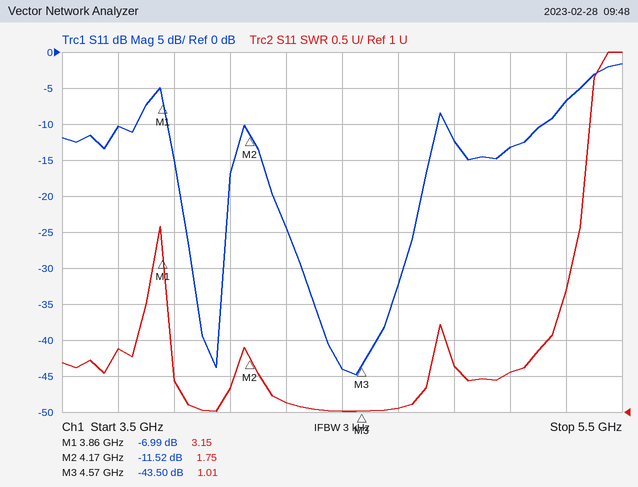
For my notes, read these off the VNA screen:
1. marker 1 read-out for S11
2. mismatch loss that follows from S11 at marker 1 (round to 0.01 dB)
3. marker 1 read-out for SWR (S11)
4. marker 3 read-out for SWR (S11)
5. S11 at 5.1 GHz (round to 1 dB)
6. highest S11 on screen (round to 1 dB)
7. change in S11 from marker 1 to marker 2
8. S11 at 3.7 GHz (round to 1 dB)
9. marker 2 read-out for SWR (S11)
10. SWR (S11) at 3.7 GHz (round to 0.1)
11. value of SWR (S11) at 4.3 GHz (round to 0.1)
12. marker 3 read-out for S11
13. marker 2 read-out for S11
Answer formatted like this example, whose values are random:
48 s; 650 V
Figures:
-6.99 dB; 0.97 dB; 3.15; 1.01; -13 dB; -2 dB; -4.53 dB; -10 dB; 1.75; 1.9; 1.1; -43.50 dB; -11.52 dB
